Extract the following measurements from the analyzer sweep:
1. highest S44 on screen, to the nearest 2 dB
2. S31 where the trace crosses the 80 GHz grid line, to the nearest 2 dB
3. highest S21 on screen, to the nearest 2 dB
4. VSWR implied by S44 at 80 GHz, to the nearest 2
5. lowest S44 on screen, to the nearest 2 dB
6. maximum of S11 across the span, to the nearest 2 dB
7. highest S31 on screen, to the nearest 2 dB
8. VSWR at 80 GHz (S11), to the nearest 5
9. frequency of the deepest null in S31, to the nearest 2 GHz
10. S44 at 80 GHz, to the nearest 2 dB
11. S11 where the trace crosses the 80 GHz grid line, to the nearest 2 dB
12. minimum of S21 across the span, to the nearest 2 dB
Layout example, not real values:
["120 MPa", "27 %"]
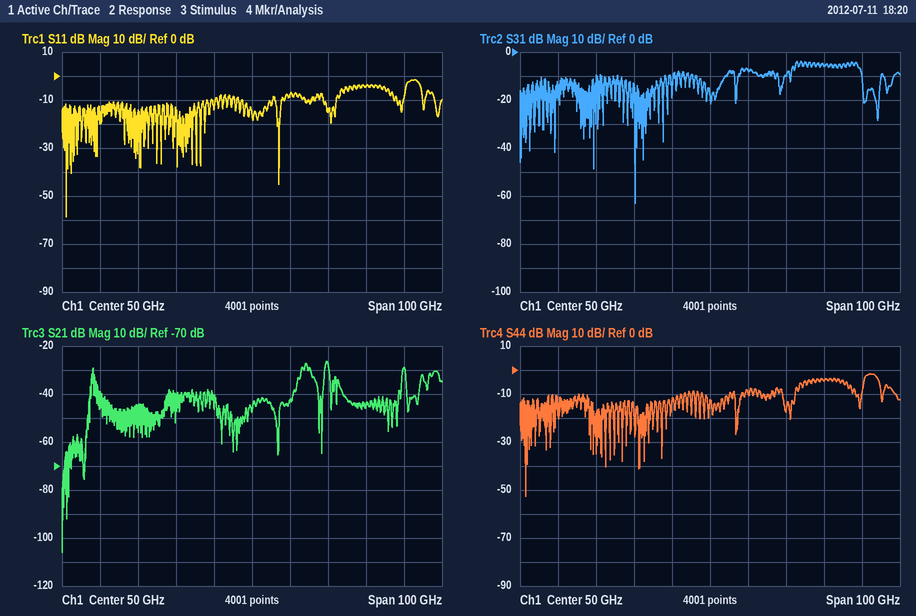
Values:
["-2 dB", "-6 dB", "-26 dB", "4", "-52 dB", "-2 dB", "-4 dB", "5", "30 GHz", "-4 dB", "-4 dB", "-106 dB"]
